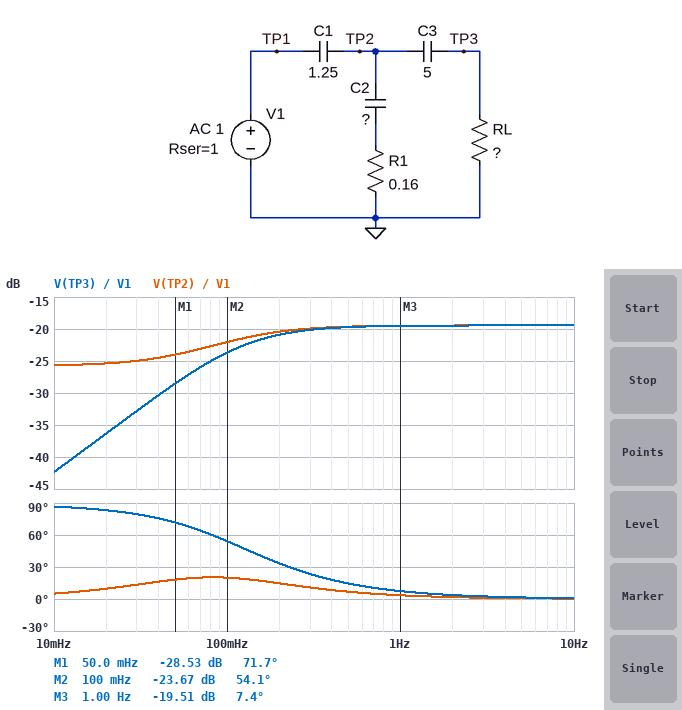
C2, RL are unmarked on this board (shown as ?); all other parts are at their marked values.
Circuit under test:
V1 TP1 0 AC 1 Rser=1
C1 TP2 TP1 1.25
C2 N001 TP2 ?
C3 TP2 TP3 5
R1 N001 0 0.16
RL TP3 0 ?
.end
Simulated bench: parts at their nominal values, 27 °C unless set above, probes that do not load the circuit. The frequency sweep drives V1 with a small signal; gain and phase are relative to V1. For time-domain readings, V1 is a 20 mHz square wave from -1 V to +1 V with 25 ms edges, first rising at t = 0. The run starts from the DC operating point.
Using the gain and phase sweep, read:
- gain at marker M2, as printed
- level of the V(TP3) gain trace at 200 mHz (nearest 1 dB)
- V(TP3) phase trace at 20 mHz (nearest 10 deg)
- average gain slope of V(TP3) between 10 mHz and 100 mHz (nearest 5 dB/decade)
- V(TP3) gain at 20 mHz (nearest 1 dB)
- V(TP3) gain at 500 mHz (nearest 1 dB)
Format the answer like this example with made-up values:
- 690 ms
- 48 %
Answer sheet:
- -23.67 dB
- -21 dB
- 80 deg
- 20 dB/decade
- -36 dB
- -20 dB
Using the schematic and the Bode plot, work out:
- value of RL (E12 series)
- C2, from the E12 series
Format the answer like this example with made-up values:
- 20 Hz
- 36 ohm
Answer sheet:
- 0.47 Ω
- 18 F
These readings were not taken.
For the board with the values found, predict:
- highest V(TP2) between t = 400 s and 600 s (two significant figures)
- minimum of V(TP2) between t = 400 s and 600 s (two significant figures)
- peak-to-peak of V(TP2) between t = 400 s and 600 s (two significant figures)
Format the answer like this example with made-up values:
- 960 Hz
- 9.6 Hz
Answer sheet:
- 210 mV
- -110 mV
- 320 mV
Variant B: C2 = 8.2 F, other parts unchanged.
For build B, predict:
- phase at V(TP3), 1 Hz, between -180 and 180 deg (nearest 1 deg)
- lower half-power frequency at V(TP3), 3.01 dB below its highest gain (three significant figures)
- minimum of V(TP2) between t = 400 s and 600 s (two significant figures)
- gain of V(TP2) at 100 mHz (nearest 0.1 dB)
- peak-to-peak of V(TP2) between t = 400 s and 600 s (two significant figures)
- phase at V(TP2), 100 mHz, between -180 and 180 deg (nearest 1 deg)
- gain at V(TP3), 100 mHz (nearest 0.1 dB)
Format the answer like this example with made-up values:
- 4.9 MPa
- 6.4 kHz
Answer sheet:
- 5 deg
- 84.9 mHz
- -40 mV
- -20.2 dB
- 250 mV
- 6 deg
- -21.8 dB
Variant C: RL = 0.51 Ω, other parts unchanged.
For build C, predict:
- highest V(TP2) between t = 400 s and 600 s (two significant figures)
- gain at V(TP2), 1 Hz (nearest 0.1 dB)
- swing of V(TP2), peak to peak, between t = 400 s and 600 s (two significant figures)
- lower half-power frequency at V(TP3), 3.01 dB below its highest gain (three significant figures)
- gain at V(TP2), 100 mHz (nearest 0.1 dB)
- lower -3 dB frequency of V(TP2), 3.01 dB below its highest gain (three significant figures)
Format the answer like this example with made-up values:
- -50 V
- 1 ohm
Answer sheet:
- 220 mV
- -19.3 dB
- 330 mV
- 124 mHz
- -21.9 dB
- 88.4 mHz
